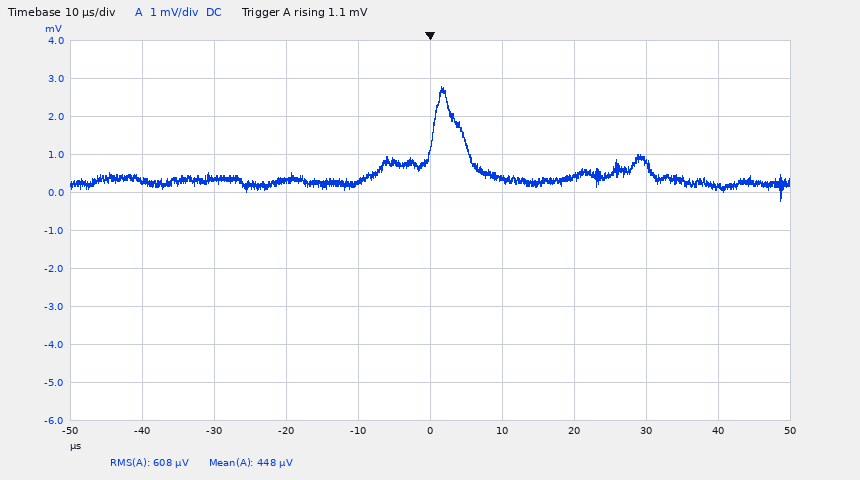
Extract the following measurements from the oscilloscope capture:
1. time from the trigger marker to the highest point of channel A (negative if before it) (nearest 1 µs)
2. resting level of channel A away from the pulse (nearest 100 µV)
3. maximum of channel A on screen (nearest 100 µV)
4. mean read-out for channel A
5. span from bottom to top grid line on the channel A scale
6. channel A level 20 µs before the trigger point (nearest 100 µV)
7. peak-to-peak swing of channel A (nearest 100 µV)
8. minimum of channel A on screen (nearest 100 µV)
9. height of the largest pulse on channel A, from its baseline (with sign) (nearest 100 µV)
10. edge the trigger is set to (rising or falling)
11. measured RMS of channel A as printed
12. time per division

+2 µs
300 µV
2.8 mV
448 µV
10 mV
300 µV
3.0 mV
-200 µV
+2.5 mV
rising
608 µV
10 µs
